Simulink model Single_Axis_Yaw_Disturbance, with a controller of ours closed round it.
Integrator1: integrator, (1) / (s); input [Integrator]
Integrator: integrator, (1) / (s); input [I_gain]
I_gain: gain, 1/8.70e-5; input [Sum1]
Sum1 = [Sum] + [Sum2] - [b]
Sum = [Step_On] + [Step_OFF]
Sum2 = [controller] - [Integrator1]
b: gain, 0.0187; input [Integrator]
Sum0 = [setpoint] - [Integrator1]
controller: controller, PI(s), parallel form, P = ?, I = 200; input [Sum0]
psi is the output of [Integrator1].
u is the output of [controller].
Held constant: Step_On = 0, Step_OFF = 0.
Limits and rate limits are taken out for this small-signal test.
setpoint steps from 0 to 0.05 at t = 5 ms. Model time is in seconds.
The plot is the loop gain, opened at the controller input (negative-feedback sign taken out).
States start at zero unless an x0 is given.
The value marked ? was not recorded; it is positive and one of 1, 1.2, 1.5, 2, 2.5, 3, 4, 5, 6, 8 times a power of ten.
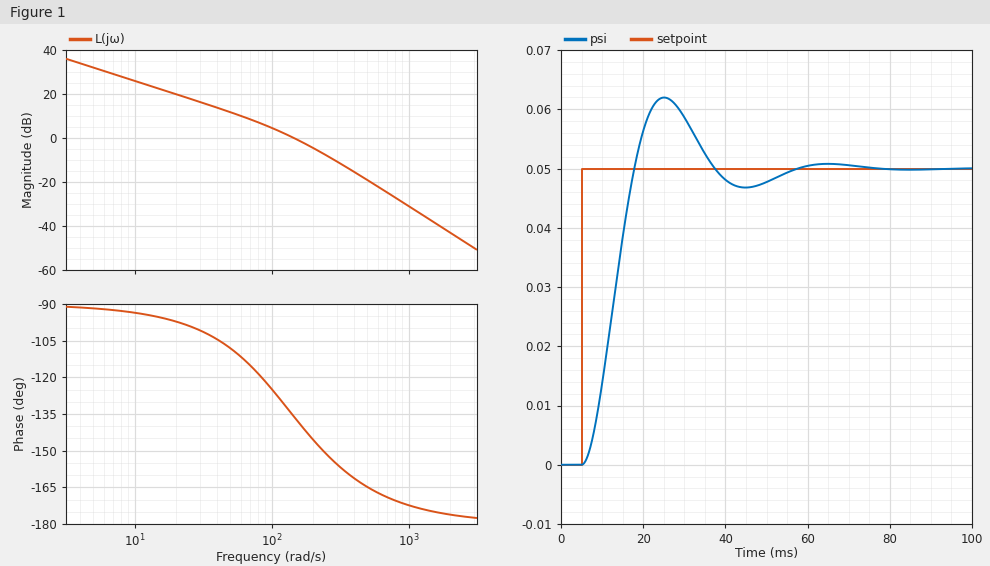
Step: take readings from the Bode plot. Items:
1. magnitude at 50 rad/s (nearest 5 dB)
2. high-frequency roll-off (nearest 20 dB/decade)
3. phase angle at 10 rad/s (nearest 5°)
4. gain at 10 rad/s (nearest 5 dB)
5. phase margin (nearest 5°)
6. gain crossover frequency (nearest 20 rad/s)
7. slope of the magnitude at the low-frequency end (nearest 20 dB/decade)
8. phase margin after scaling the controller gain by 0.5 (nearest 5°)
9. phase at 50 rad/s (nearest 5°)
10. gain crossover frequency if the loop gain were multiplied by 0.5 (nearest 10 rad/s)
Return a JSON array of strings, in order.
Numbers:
["10 dB", "-40 dB/decade", "-95°", "25 dB", "45°", "140 rad/s", "-20 dB/decade", "60°", "-110°", "90 rad/s"]
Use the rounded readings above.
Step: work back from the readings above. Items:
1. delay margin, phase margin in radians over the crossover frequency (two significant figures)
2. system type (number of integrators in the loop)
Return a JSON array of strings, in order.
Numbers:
["0.0056 s", "1"]
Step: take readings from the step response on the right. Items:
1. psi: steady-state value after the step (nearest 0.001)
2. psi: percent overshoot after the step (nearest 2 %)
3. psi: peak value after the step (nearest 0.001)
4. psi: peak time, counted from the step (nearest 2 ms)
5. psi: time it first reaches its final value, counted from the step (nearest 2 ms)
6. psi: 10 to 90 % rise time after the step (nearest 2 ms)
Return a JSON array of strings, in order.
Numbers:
["0.050", "24 %", "0.062", "20 ms", "12 ms", "8 ms"]
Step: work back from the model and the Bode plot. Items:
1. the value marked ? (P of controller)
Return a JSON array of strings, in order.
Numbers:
["2.5"]
